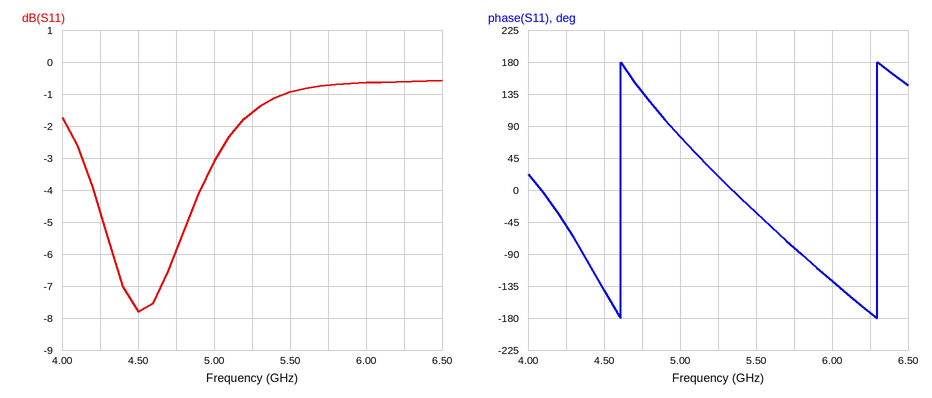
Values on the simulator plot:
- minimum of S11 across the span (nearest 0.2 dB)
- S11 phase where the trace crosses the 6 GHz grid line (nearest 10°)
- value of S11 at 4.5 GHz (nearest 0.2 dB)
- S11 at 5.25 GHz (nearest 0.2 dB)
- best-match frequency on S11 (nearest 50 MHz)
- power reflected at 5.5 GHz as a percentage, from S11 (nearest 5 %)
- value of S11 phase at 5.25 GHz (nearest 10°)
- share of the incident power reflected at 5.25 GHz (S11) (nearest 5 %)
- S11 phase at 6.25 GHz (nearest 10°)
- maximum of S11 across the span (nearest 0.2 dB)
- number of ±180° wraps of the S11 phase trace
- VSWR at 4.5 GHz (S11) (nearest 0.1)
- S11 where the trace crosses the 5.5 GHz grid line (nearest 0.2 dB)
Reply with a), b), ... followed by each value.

a) -7.8 dB
b) -130°
c) -7.8 dB
d) -1.6 dB
e) 4.50 GHz
f) 80 %
g) 20°
h) 70 %
i) -170°
j) -0.6 dB
k) 2
l) 2.4
m) -1.0 dB
